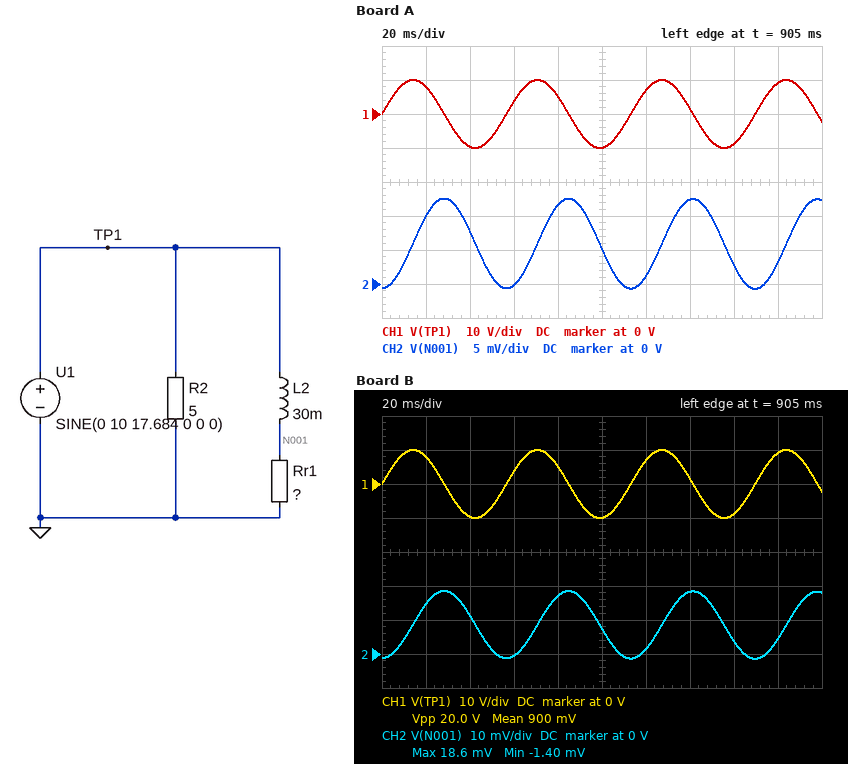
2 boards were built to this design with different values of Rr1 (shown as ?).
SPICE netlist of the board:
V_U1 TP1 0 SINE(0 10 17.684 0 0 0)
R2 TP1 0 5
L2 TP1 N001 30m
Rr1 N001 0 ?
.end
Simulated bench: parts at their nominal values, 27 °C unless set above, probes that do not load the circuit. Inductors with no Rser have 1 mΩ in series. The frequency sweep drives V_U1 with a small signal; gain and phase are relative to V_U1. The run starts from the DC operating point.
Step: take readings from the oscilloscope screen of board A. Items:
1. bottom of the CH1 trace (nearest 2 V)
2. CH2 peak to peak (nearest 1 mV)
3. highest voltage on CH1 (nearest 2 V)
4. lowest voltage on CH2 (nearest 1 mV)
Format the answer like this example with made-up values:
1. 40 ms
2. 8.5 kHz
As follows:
1. -10 V
2. 13 mV
3. 10 V
4. -1 mV
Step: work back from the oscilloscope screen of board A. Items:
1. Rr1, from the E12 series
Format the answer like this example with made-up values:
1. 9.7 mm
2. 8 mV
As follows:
1. 2.2 mΩ
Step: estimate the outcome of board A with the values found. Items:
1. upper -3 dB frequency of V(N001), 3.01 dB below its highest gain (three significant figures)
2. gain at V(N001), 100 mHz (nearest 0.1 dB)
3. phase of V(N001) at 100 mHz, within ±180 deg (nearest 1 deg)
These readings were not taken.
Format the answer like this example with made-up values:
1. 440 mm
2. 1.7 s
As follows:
1. 17.0 mHz
2. -18.8 dB
3. -80 deg
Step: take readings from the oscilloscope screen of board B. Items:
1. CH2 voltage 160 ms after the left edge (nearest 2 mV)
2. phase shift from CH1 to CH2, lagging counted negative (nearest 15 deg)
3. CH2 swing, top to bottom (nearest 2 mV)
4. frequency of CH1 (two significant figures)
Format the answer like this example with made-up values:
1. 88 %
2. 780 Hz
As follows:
1. 4 mV
2. -90 deg
3. 20 mV
4. 18 Hz
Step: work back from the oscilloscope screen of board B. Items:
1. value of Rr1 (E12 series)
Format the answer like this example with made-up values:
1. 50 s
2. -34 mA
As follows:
1. 3.3 mΩ
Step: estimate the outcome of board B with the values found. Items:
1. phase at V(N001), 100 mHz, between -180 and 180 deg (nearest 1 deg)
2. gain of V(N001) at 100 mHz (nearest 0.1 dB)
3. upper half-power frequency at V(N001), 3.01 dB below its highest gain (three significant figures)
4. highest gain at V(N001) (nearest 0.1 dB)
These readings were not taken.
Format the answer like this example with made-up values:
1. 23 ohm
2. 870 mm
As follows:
1. -77 deg
2. -15.4 dB
3. 22.8 mHz
4. -2.3 dB
